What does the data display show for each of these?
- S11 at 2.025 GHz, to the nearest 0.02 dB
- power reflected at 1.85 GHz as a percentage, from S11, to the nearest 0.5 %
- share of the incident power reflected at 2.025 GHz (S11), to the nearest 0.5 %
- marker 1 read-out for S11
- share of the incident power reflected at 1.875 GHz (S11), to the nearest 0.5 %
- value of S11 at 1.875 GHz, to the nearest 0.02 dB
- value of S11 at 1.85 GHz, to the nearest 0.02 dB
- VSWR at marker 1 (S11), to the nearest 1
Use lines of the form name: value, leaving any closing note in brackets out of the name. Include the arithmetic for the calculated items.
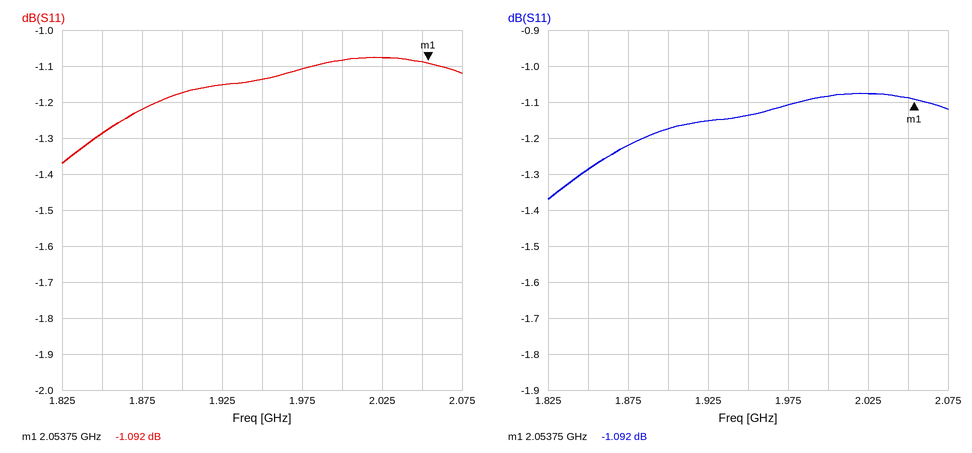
S11 at 2.025 GHz, to the nearest 0.02 dB: -1.08 dB
power reflected at 1.85 GHz as a percentage, from S11, to the nearest 0.5 %: 10^(-1.28/10) ≈ 74.5 %
share of the incident power reflected at 2.025 GHz (S11), to the nearest 0.5 %: 10^(-1.08/10) ≈ 78.0 %
marker 1 read-out for S11: -1.092 dB
share of the incident power reflected at 1.875 GHz (S11), to the nearest 0.5 %: 10^(-1.22/10) ≈ 75.5 %
value of S11 at 1.875 GHz, to the nearest 0.02 dB: -1.22 dB
value of S11 at 1.85 GHz, to the nearest 0.02 dB: -1.28 dB
VSWR at marker 1 (S11), to the nearest 1: (1 + 0.8819)/(1 − 0.8819) ≈ 16
